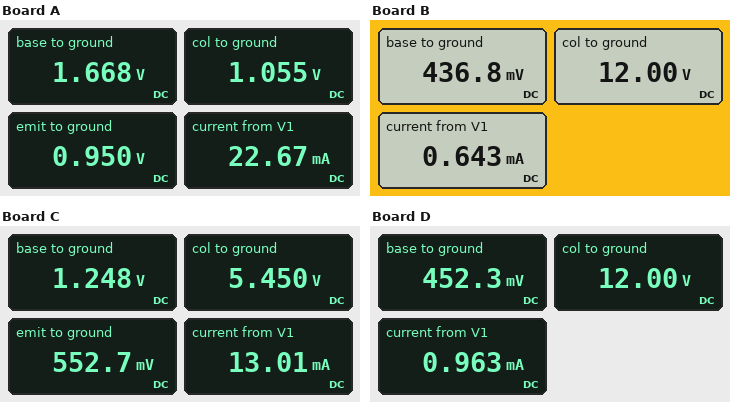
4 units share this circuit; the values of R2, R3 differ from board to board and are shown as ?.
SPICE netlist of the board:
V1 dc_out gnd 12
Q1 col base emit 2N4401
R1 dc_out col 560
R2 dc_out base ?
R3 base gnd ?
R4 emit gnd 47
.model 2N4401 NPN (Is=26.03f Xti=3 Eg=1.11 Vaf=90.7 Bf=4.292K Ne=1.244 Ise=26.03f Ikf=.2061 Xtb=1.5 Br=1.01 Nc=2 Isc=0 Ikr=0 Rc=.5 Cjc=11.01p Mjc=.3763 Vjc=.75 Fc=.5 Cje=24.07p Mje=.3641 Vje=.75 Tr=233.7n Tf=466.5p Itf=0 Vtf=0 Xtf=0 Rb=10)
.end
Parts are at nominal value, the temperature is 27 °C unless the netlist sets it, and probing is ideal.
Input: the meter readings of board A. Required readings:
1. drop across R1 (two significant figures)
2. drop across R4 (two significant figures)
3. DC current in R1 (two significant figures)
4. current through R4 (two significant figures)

11 V
950 mV
20 mA
20 mA
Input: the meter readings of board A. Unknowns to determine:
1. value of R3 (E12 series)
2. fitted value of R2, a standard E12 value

680 Ω
3.3 kΩ
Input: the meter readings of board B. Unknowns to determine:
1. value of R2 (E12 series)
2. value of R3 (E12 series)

18 kΩ
680 Ω
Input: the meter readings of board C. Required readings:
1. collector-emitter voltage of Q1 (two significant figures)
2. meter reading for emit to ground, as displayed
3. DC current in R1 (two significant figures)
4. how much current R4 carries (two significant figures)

4.9 V
552.7 mV
12 mA
12 mA
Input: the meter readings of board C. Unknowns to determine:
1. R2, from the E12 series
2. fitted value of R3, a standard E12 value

8.2 kΩ
1 kΩ
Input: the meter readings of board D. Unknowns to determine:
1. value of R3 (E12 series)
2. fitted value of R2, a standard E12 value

470 Ω
12 kΩ
